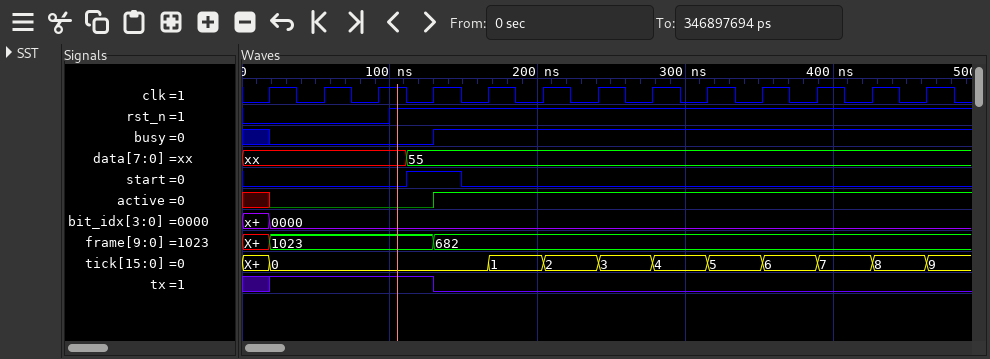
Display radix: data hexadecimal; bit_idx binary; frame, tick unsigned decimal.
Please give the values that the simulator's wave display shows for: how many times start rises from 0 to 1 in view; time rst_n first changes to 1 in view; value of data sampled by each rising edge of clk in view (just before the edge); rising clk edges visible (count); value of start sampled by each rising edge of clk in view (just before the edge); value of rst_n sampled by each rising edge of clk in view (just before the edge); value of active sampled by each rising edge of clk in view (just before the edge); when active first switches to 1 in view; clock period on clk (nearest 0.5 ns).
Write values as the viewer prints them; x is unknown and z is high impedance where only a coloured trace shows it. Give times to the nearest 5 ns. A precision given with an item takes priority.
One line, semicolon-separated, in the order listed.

1; 100 ns; xx, xx, xx, 55, 55, 55, 55, 55, 55, 55, 55, 55, 55; 13; 0 0 0 1 0 0 0 0 0 0 0 0 0; 0 0 0 1 1 1 1 1 1 1 1 1 1; x 0 0 0 1 1 1 1 1 1 1 1 1; 130 ns; 37 ns
